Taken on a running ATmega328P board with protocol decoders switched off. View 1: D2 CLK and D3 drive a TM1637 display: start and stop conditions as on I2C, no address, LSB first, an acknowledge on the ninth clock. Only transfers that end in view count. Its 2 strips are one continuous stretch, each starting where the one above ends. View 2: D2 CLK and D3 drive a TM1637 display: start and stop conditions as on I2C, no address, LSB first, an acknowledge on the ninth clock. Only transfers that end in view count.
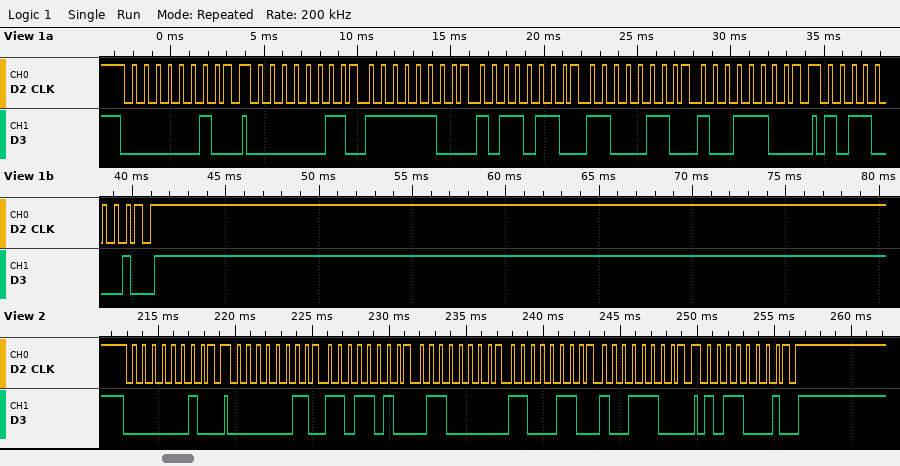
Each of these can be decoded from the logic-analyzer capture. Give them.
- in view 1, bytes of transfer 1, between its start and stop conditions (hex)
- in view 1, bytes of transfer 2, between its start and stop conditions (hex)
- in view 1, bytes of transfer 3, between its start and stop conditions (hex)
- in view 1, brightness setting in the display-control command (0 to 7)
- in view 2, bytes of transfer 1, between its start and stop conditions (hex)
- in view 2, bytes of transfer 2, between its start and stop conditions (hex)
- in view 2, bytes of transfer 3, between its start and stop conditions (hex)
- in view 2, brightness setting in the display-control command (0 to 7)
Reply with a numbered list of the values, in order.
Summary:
1. 40
2. C0 3F 6D 63 39
3. 8D
4. 5
5. 40
6. C0 5B 06 63 39
7. 8D
8. 5
